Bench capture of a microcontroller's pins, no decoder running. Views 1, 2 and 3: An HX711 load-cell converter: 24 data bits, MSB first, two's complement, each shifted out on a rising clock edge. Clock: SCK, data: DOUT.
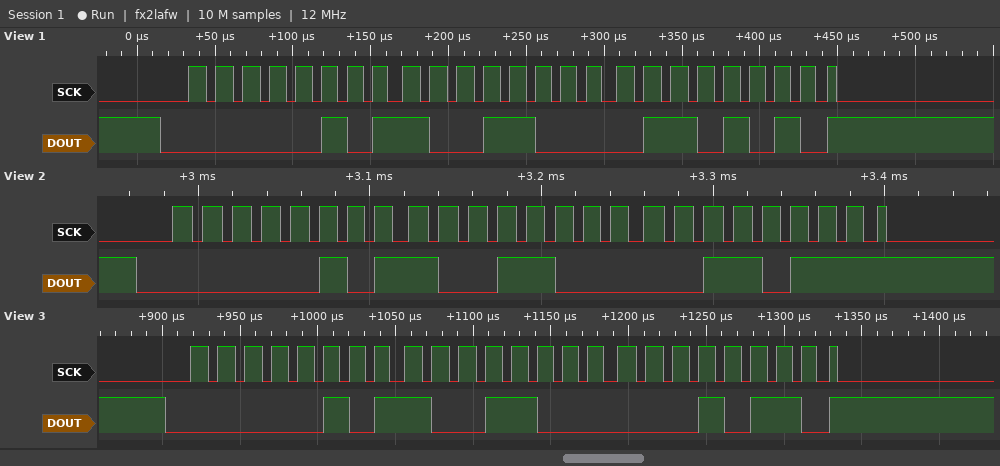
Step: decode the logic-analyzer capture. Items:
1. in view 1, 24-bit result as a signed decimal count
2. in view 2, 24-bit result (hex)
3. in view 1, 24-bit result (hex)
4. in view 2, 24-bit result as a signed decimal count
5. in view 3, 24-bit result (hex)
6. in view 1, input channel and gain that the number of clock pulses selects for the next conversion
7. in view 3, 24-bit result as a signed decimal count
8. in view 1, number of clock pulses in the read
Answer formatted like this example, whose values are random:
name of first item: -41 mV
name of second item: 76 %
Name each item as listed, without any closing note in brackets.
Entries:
in view 1, 24-bit result as a signed decimal count: 366698
in view 2, 24-bit result: 0x059837
in view 1, 24-bit result: 0x05986A
in view 2, 24-bit result as a signed decimal count: 366647
in view 3, 24-bit result: 0x059816
in view 1, input channel and gain that the number of clock pulses selects for the next conversion: channel A, gain 128
in view 3, 24-bit result as a signed decimal count: 366614
in view 1, number of clock pulses in the read: 25
